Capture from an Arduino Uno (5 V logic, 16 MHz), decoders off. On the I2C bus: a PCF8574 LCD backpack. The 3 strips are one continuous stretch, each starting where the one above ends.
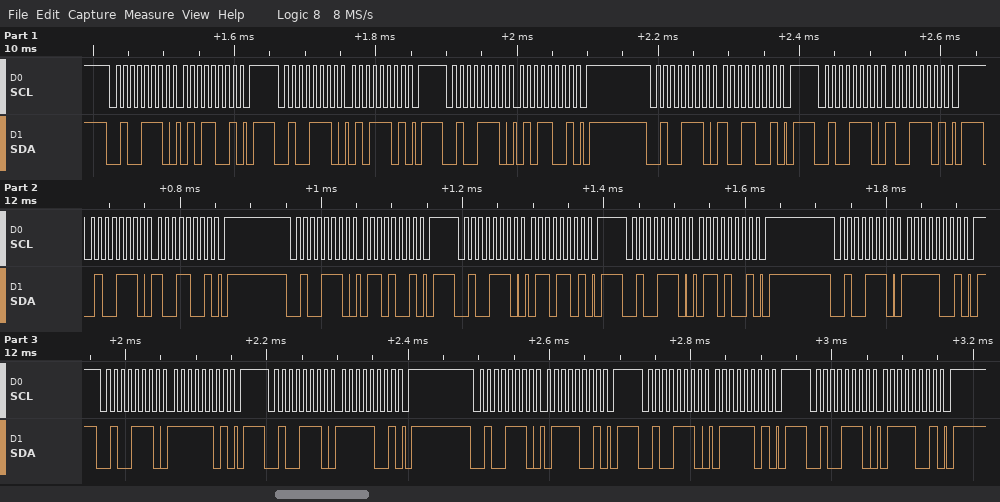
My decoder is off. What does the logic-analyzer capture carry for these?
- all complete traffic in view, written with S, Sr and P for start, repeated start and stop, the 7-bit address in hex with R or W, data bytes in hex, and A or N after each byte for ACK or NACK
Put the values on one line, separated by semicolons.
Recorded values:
S 27W A 59 A P S 27W A 5D A P S 27W A 59 A P S 27W A 99 A P S 27W A 9D A P S 27W A 99 A P S 27W A 69 A P S 27W A 6D A P S 27W A 69 A P S 27W A F9 A P S 27W A FD A P S 27W A F9 A P S 27W A 79 A P S 27W A 7D A P S 27W A 79 A P
